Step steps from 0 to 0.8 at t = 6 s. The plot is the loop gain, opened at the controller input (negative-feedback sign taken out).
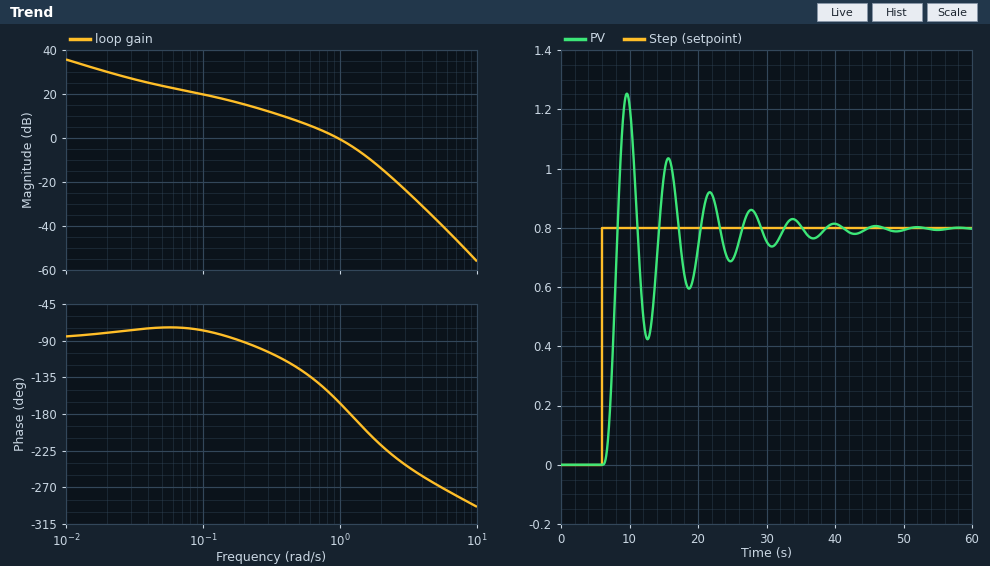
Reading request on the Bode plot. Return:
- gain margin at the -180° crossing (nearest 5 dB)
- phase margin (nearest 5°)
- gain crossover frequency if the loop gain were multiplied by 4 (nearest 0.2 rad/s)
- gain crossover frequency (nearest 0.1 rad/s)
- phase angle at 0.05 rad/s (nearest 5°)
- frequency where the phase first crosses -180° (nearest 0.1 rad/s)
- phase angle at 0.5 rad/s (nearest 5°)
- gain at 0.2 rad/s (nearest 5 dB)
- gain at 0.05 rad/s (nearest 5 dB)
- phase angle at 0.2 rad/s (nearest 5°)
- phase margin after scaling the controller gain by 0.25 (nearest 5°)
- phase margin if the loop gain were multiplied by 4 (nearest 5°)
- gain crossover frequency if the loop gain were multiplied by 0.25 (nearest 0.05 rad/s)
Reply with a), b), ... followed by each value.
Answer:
a) 5 dB
b) 15°
c) 1.8 rad/s
d) 1.0 rad/s
e) -75°
f) 1.2 rad/s
g) -125°
h) 15 dB
i) 25 dB
j) -90°
k) 75°
l) -35°
m) 0.30 rad/s
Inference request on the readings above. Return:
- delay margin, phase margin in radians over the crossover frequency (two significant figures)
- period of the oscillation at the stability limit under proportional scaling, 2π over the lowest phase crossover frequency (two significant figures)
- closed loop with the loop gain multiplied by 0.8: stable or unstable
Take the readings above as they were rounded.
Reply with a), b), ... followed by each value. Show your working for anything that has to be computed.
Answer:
a) 15 × π / 180 / 1 = 0.26 s
b) 2π / 1.2 = 5.2 s
c) stable
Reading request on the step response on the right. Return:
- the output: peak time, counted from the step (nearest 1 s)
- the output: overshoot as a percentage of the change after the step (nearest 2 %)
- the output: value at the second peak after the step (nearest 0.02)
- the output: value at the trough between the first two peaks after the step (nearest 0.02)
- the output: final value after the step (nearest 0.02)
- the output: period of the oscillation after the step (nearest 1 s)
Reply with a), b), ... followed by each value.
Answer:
a) 4 s
b) 56 %
c) 1.04
d) 0.42
e) 0.80
f) 6 s
